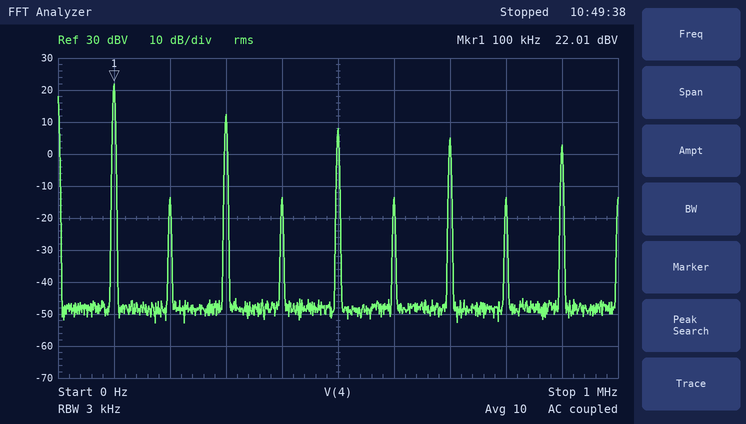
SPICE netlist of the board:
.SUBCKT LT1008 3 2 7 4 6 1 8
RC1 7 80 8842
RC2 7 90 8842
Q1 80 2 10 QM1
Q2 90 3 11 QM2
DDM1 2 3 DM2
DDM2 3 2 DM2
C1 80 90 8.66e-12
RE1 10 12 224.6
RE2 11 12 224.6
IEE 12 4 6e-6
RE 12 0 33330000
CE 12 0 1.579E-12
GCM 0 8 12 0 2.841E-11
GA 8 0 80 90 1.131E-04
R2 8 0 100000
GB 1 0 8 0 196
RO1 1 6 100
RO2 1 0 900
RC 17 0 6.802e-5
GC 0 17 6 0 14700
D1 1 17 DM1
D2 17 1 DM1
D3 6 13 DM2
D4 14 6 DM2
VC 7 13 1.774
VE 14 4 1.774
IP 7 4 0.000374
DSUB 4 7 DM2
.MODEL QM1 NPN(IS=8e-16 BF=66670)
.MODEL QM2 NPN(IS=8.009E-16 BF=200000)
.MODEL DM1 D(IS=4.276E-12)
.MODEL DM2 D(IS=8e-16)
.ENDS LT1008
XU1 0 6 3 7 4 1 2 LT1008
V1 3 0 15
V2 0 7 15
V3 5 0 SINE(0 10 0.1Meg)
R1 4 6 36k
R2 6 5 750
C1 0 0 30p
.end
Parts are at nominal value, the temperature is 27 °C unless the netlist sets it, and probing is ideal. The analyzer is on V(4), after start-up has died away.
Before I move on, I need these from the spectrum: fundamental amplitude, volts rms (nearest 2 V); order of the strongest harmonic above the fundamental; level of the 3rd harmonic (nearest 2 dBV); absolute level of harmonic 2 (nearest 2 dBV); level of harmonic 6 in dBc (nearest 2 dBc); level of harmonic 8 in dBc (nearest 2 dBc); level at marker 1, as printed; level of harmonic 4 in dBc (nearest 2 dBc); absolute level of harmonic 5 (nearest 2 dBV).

12 V
3
12 dBV
-14 dBV
-36 dBc
-36 dBc
22.01 dBV
-36 dBc
8 dBV
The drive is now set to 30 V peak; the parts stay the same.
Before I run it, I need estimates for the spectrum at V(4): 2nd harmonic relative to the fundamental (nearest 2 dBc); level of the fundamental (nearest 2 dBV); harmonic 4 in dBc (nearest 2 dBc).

-26 dBc
22 dBV
-26 dBc
